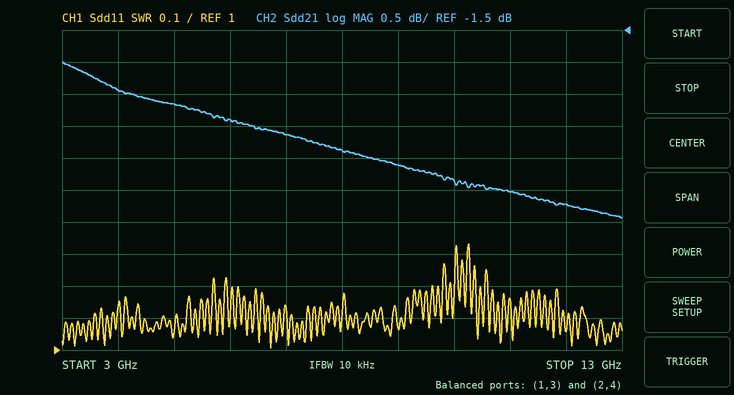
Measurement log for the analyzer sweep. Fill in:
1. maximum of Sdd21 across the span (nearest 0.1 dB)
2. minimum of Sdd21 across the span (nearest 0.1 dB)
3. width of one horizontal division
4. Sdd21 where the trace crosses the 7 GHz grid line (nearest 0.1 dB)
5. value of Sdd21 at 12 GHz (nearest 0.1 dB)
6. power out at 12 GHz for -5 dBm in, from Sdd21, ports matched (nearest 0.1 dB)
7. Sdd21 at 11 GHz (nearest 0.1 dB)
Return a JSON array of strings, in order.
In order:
["-2.0 dB", "-4.4 dB", "1 GHz", "-3.1 dB", "-4.2 dB", "-9.2 dBm", "-4.0 dB"]
